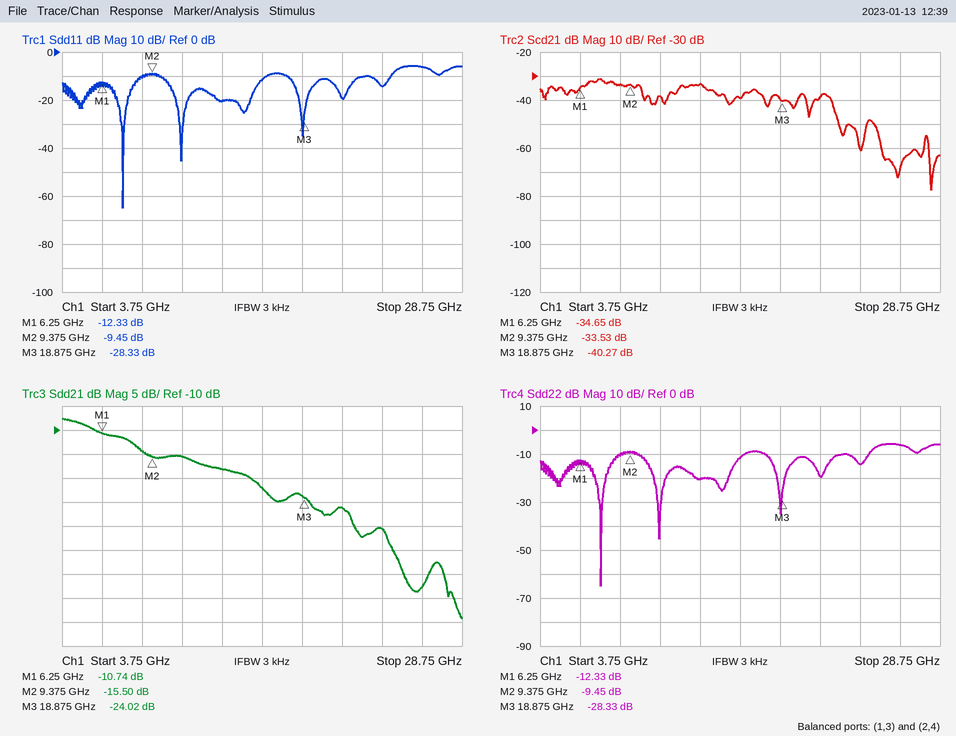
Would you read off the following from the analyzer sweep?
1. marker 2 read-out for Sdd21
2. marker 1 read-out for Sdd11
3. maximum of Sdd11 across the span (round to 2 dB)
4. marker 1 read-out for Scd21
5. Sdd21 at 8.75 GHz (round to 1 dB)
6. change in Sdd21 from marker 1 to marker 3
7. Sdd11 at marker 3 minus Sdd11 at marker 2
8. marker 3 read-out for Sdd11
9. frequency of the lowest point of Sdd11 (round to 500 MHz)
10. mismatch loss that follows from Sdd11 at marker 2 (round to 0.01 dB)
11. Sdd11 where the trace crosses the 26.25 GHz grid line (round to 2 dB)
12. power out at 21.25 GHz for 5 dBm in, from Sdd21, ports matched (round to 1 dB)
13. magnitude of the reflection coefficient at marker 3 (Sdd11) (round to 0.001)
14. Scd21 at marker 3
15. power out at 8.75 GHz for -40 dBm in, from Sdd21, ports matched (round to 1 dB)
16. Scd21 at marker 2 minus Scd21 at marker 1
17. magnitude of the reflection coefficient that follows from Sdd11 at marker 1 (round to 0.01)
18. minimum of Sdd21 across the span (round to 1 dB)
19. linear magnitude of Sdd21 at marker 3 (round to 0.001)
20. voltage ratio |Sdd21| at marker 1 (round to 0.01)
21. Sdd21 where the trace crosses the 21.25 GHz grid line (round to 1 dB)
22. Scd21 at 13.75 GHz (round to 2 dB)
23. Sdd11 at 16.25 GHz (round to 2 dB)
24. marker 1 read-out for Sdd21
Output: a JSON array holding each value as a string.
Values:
["-15.50 dB", "-12.33 dB", "-6 dB", "-34.65 dB", "-14 dB", "-13.28 dB", "-18.88 dB", "-28.33 dB", "7.5 GHz", "0.52 dB", "-6 dB", "-21 dBm", "0.038", "-40.27 dB", "-54 dBm", "1.12 dB", "0.24", "-49 dB", "0.063", "0.29", "-26 dB", "-34 dB", "-12 dB", "-10.74 dB"]
